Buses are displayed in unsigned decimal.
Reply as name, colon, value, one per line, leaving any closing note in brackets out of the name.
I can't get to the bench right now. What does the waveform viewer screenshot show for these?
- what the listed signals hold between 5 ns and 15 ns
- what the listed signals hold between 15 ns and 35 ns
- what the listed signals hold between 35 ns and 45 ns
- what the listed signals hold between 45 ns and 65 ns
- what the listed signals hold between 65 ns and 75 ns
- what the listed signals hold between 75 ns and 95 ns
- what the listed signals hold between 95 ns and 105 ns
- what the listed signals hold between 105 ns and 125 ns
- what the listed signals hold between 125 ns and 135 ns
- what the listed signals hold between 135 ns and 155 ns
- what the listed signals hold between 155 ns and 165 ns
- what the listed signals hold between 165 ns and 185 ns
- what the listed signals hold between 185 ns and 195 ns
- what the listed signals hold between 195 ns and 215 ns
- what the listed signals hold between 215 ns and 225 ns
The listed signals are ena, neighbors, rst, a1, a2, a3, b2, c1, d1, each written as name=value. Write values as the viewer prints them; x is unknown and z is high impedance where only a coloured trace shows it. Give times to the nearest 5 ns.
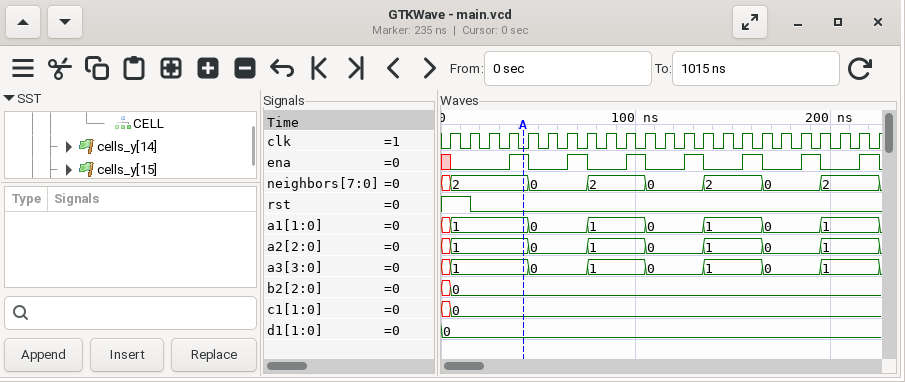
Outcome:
what the listed signals hold between 5 ns and 15 ns: ena=0, neighbors=2, rst=1, a1=1, a2=1, a3=1, b2=0, c1=0, d1=0
what the listed signals hold between 15 ns and 35 ns: ena=0, neighbors=2, rst=0, a1=1, a2=1, a3=1, b2=0, c1=0, d1=0
what the listed signals hold between 35 ns and 45 ns: ena=1, neighbors=2, rst=0, a1=1, a2=1, a3=1, b2=0, c1=0, d1=0
what the listed signals hold between 45 ns and 65 ns: ena=0, neighbors=0, rst=0, a1=0, a2=0, a3=0, b2=0, c1=0, d1=0
what the listed signals hold between 65 ns and 75 ns: ena=1, neighbors=0, rst=0, a1=0, a2=0, a3=0, b2=0, c1=0, d1=0
what the listed signals hold between 75 ns and 95 ns: ena=0, neighbors=2, rst=0, a1=1, a2=1, a3=1, b2=0, c1=0, d1=0
what the listed signals hold between 95 ns and 105 ns: ena=1, neighbors=2, rst=0, a1=1, a2=1, a3=1, b2=0, c1=0, d1=0
what the listed signals hold between 105 ns and 125 ns: ena=0, neighbors=0, rst=0, a1=0, a2=0, a3=0, b2=0, c1=0, d1=0
what the listed signals hold between 125 ns and 135 ns: ena=1, neighbors=0, rst=0, a1=0, a2=0, a3=0, b2=0, c1=0, d1=0
what the listed signals hold between 135 ns and 155 ns: ena=0, neighbors=2, rst=0, a1=1, a2=1, a3=1, b2=0, c1=0, d1=0
what the listed signals hold between 155 ns and 165 ns: ena=1, neighbors=2, rst=0, a1=1, a2=1, a3=1, b2=0, c1=0, d1=0
what the listed signals hold between 165 ns and 185 ns: ena=0, neighbors=0, rst=0, a1=0, a2=0, a3=0, b2=0, c1=0, d1=0
what the listed signals hold between 185 ns and 195 ns: ena=1, neighbors=0, rst=0, a1=0, a2=0, a3=0, b2=0, c1=0, d1=0
what the listed signals hold between 195 ns and 215 ns: ena=0, neighbors=2, rst=0, a1=1, a2=1, a3=1, b2=0, c1=0, d1=0
what the listed signals hold between 215 ns and 225 ns: ena=1, neighbors=2, rst=0, a1=1, a2=1, a3=1, b2=0, c1=0, d1=0
